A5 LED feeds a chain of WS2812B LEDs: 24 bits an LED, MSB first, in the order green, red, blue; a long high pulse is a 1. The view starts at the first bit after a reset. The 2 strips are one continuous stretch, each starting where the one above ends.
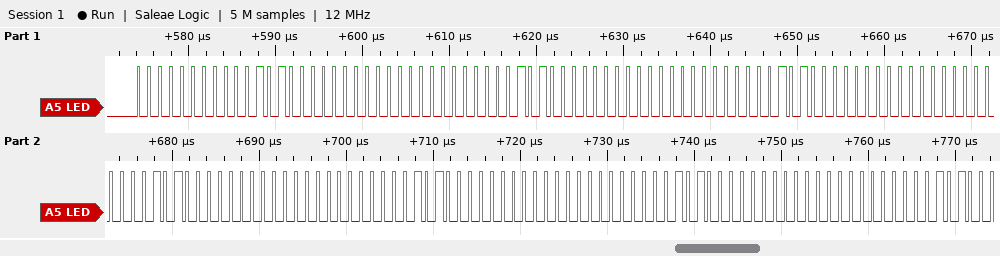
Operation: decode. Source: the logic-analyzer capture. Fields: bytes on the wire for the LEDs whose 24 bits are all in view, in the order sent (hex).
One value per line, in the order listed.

00 14 00 00 14 00 00 14 00 00 14 00 00 14 00 00 14 00
